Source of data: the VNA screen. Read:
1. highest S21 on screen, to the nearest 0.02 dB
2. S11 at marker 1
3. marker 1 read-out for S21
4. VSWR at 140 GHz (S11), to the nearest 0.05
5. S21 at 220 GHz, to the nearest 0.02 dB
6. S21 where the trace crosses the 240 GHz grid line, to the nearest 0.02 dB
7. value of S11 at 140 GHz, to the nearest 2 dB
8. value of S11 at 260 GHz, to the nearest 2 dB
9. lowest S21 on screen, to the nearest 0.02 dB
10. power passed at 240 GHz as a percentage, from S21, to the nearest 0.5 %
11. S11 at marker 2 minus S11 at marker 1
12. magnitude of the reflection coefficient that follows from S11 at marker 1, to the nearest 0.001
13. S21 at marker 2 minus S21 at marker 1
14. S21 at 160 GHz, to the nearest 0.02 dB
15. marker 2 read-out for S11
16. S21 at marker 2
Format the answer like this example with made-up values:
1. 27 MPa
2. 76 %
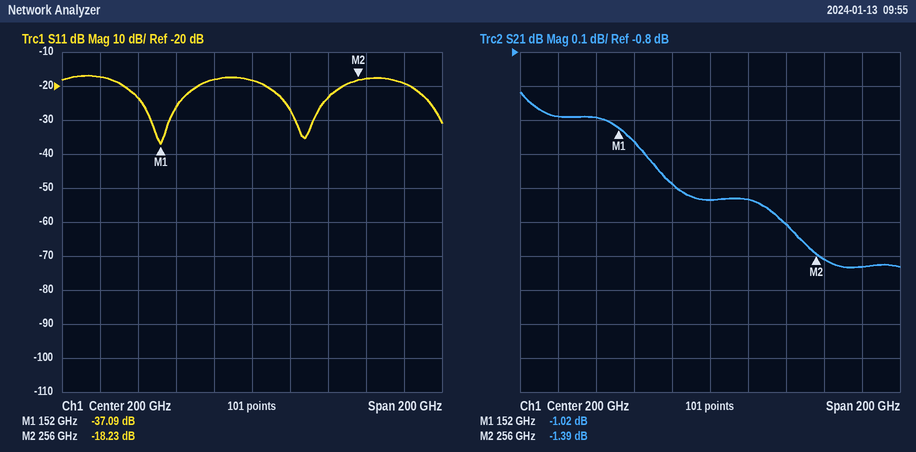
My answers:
1. -0.92 dB
2. -37.09 dB
3. -1.02 dB
4. 1.15
5. -1.24 dB
6. -1.30 dB
7. -24 dB
8. -18 dB
9. -1.44 dB
10. 74.0 %
11. 18.86 dB
12. 0.014
13. -0.37 dB
14. -1.06 dB
15. -18.23 dB
16. -1.39 dB
